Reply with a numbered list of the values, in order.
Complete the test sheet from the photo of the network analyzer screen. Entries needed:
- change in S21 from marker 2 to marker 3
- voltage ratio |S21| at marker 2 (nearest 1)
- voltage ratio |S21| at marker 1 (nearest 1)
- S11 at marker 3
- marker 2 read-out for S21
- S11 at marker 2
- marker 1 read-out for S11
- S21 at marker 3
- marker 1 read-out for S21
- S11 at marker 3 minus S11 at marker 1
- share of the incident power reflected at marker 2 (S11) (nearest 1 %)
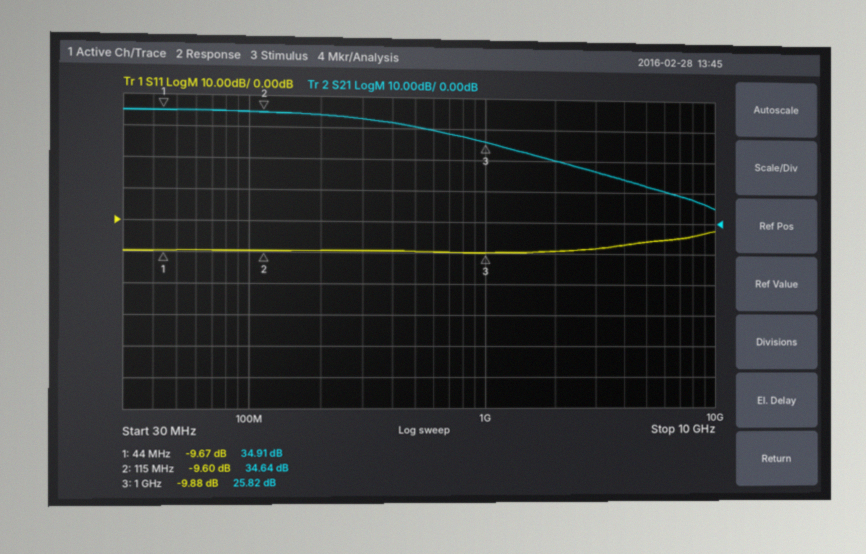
1. -8.82 dB
2. 54
3. 56
4. -9.88 dB
5. 34.64 dB
6. -9.60 dB
7. -9.67 dB
8. 25.82 dB
9. 34.91 dB
10. -0.21 dB
11. 11 %
